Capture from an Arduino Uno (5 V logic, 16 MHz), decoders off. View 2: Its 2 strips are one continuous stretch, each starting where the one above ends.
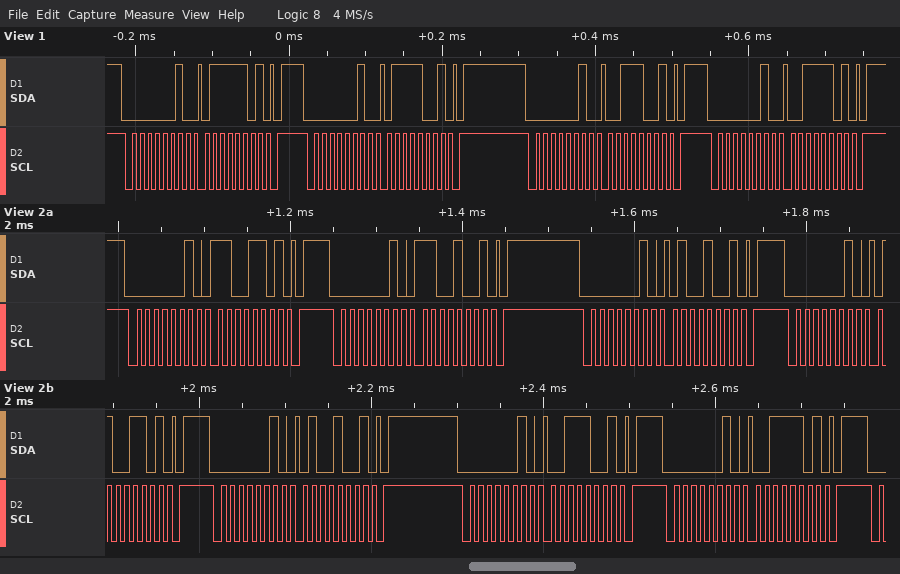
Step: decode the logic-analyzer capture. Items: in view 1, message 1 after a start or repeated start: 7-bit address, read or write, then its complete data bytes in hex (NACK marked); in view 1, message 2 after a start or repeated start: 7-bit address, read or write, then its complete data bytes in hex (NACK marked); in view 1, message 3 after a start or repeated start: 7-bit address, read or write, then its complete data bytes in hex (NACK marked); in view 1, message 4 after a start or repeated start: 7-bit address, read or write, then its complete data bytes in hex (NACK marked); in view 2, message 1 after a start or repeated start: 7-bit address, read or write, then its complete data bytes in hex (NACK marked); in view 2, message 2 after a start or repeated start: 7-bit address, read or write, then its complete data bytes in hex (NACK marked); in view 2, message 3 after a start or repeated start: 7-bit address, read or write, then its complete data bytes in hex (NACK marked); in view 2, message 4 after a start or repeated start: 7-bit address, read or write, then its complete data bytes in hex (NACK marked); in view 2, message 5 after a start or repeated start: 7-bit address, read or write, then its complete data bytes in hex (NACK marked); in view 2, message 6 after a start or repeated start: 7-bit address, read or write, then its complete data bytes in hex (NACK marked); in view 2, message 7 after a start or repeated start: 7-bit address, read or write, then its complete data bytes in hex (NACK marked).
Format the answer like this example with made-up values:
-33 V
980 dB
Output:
0x01 write: 7D
0x01 write: 79
0x01 write: 39
0x01 write: 3D
0x01 write: CD
0x01 write: C9
0x01 write: 49
0x01 write: 4D
0x01 write: 49
0x01 write: 39
0x01 write: 3D
